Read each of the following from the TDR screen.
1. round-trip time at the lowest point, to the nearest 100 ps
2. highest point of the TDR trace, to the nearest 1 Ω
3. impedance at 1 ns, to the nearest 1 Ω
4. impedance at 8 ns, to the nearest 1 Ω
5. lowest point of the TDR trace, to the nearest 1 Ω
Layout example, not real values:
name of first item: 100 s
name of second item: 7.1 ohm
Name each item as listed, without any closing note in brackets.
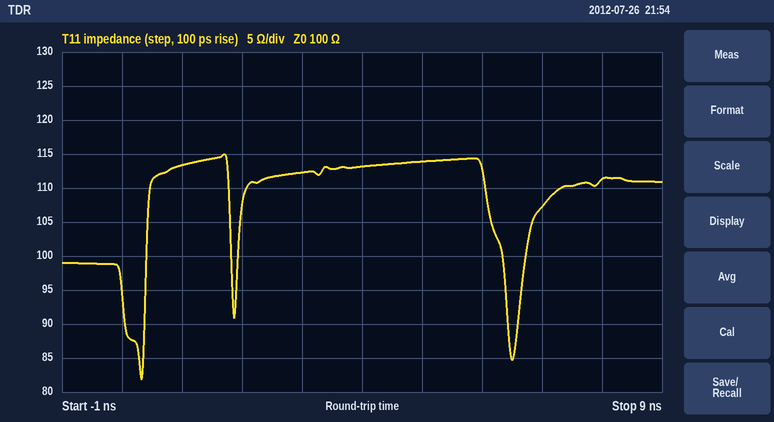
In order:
round-trip time at the lowest point, to the nearest 100 ps: 300 ps
highest point of the TDR trace, to the nearest 1 Ω: 115 Ω
impedance at 1 ns, to the nearest 1 Ω: 113 Ω
impedance at 8 ns, to the nearest 1 Ω: 111 Ω
lowest point of the TDR trace, to the nearest 1 Ω: 82 Ω
